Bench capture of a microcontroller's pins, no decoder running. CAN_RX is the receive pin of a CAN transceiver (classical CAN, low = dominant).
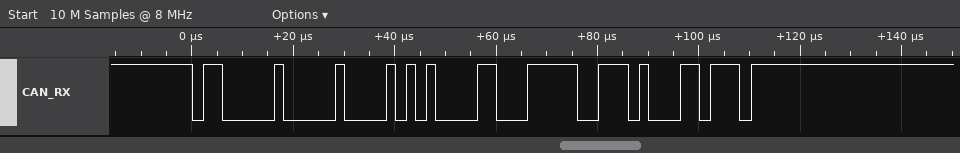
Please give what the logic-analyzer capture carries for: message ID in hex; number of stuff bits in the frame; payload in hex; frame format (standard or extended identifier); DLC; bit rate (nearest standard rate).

0x600
3
A1 8F
standard
2
500 kbit/s
